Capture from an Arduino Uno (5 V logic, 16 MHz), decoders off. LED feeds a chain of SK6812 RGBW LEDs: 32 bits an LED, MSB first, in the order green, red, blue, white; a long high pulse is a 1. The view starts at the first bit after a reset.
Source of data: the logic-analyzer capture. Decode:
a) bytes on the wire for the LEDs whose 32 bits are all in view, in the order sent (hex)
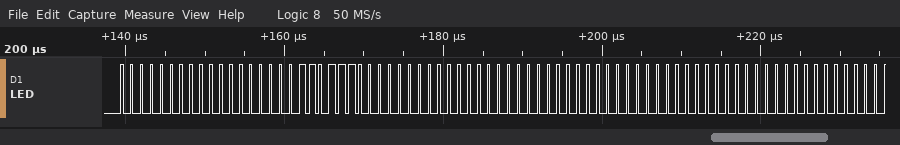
00 00 37 00 00 00 00 00
